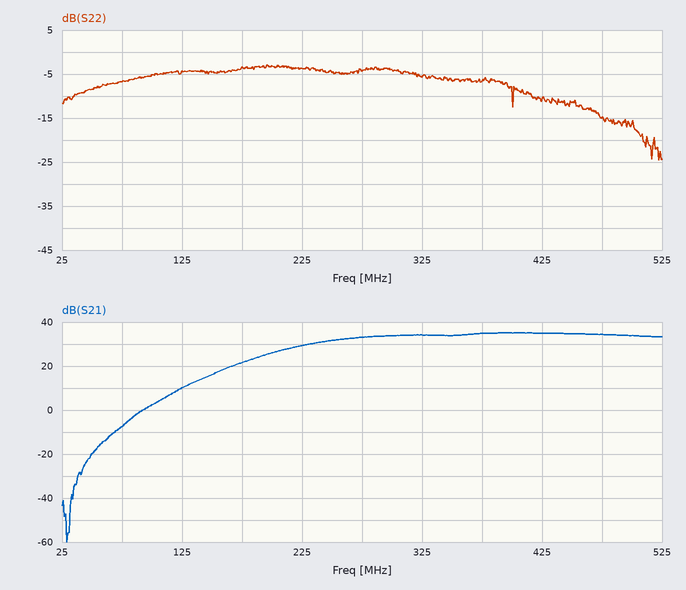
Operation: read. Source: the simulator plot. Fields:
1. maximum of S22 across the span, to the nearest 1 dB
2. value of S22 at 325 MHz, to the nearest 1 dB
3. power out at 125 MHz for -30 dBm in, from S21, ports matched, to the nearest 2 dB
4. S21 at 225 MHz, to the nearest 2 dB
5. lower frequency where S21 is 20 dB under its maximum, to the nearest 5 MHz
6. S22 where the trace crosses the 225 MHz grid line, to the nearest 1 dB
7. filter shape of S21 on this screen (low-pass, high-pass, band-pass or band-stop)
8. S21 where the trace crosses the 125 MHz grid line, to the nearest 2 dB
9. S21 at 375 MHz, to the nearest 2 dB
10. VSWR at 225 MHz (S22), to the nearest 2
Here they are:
-3 dB
-6 dB
-20 dBm
30 dB
145 MHz
-4 dB
high-pass
10 dB
34 dB
4
